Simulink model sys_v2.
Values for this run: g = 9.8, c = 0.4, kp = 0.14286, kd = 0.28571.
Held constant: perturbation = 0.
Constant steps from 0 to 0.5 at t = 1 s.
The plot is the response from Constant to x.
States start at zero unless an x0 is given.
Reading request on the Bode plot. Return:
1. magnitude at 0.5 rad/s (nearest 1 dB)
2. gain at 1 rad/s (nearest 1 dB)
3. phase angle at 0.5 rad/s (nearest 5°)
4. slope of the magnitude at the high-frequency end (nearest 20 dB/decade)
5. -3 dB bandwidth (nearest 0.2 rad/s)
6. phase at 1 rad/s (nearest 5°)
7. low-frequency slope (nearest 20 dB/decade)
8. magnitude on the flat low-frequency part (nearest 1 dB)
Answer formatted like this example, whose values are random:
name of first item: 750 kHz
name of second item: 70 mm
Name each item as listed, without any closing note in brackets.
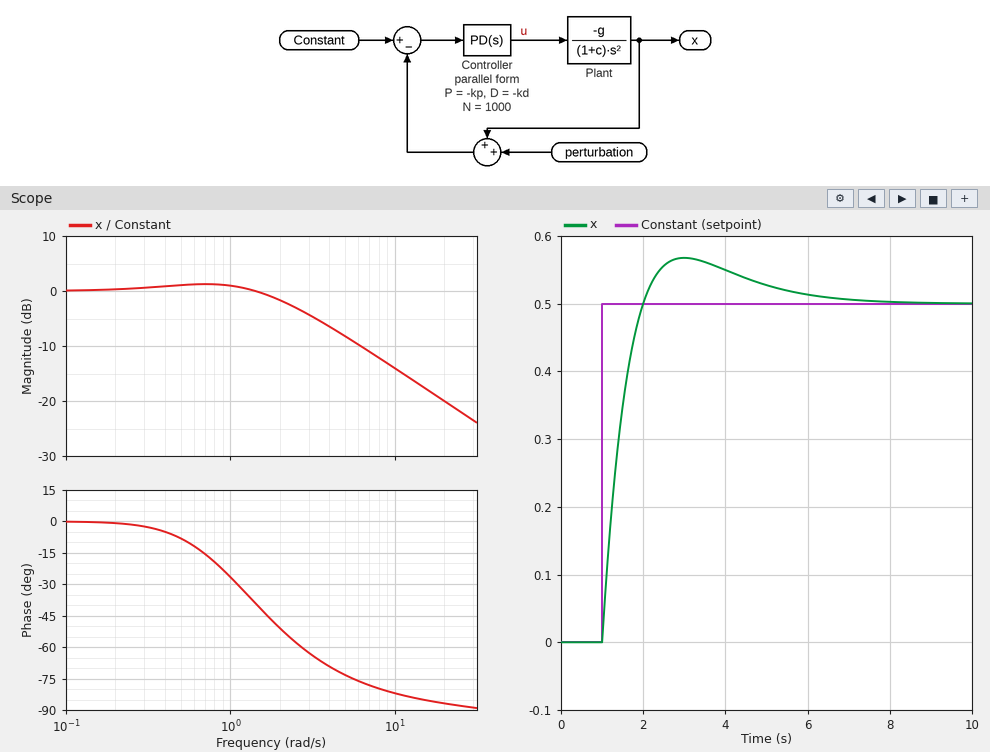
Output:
magnitude at 0.5 rad/s: 1 dB
gain at 1 rad/s: 1 dB
phase angle at 0.5 rad/s: -10°
slope of the magnitude at the high-frequency end: -20 dB/decade
-3 dB bandwidth: 2.4 rad/s
phase at 1 rad/s: -25°
low-frequency slope: 0 dB/decade
magnitude on the flat low-frequency part: 0 dB
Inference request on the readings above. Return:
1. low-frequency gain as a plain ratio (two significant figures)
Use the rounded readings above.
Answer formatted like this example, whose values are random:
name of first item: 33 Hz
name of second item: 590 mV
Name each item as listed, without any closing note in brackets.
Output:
low-frequency gain as a plain ratio: 1.0
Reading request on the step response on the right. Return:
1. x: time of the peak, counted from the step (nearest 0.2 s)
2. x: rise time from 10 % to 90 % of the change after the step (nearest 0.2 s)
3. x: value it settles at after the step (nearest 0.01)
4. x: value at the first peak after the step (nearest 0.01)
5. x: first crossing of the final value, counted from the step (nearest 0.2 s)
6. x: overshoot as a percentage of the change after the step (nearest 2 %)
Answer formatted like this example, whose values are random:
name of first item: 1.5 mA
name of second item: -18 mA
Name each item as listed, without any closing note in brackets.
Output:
x: time of the peak, counted from the step: 2.0 s
x: rise time from 10 % to 90 % of the change after the step: 0.8 s
x: value it settles at after the step: 0.50
x: value at the first peak after the step: 0.57
x: first crossing of the final value, counted from the step: 1.0 s
x: overshoot as a percentage of the change after the step: 14 %
